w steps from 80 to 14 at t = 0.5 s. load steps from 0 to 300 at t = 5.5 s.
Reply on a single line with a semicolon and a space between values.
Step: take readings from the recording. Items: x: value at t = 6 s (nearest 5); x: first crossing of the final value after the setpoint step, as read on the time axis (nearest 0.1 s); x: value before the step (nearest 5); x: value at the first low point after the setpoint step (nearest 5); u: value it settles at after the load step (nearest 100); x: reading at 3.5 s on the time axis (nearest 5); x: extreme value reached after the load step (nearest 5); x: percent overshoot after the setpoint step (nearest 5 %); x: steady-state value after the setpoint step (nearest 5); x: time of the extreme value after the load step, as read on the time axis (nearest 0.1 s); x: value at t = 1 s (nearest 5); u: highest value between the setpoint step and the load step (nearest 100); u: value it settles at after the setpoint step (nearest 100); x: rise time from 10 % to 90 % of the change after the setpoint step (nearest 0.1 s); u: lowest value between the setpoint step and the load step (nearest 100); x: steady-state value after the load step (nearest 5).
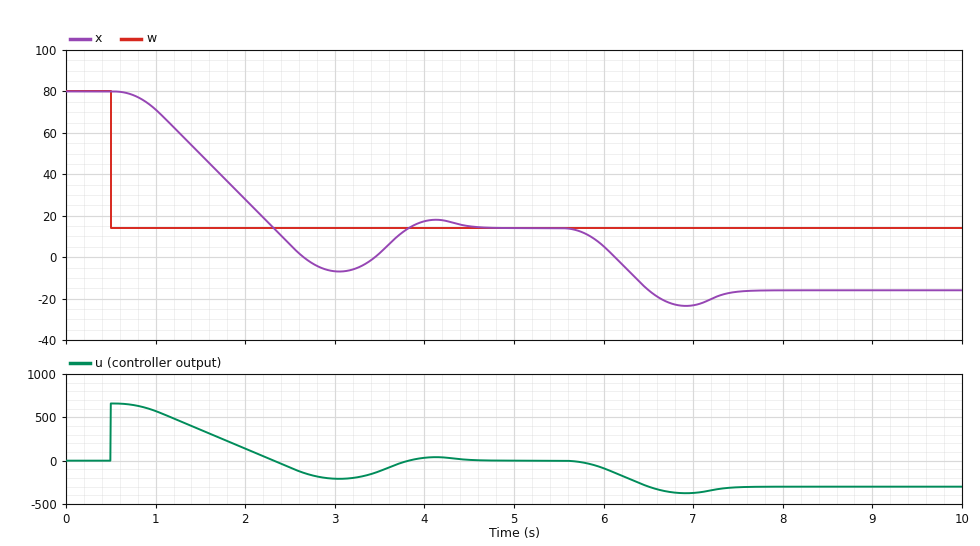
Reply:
5; 2.3 s; 80; -5; -300; 0; -25; 30 %; 15; 6.9 s; 70; 700; 0; 1.2 s; -200; -15
